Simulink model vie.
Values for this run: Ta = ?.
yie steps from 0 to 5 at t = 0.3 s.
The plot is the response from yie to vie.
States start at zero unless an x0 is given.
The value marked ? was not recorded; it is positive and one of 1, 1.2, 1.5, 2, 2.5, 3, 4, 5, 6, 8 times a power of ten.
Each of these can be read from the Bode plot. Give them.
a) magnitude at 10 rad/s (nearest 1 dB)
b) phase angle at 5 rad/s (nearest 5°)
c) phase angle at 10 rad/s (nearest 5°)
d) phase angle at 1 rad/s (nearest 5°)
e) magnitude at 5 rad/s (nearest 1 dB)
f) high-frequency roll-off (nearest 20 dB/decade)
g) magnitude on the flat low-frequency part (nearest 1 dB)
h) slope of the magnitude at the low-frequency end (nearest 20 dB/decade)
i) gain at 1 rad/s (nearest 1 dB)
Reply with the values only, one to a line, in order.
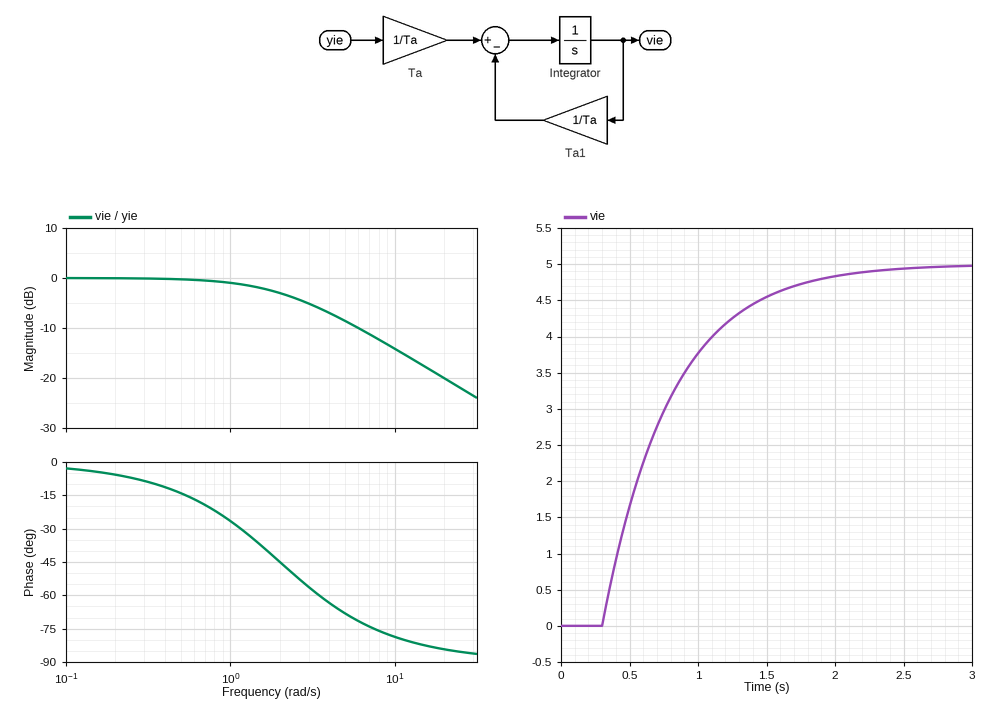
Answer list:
-14 dB
-70°
-80°
-25°
-9 dB
-20 dB/decade
0 dB
0 dB/decade
-1 dB
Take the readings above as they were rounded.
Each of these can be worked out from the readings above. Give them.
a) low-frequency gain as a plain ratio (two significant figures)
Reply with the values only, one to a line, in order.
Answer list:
1.0
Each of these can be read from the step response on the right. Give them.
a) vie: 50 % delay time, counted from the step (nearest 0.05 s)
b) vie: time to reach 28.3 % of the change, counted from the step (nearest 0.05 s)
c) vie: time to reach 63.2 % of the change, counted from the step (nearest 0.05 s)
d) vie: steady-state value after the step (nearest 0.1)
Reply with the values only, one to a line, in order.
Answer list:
0.35 s
0.15 s
0.50 s
5.0
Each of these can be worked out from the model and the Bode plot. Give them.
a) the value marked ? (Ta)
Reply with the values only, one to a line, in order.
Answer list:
0.5
